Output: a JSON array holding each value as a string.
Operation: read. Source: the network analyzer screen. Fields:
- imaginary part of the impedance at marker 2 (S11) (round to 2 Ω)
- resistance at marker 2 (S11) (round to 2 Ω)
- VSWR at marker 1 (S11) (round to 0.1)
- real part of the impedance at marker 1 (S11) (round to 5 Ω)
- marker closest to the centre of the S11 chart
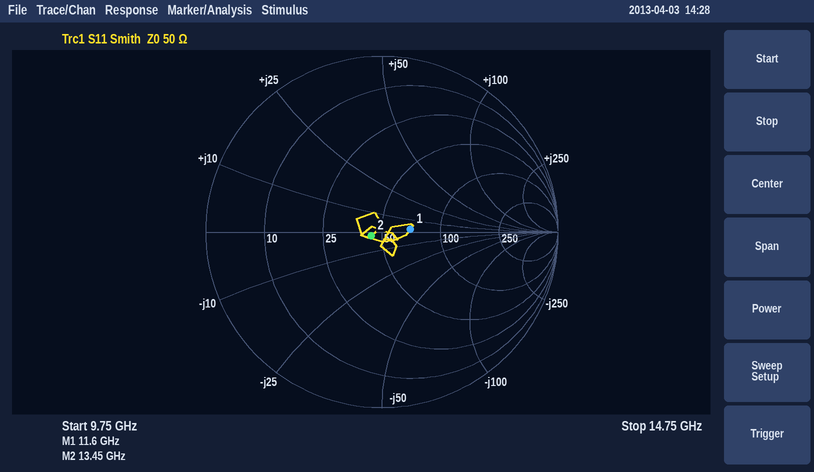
["-2 Ω", "44 Ω", "1.4", "70 Ω", "marker 2"]
